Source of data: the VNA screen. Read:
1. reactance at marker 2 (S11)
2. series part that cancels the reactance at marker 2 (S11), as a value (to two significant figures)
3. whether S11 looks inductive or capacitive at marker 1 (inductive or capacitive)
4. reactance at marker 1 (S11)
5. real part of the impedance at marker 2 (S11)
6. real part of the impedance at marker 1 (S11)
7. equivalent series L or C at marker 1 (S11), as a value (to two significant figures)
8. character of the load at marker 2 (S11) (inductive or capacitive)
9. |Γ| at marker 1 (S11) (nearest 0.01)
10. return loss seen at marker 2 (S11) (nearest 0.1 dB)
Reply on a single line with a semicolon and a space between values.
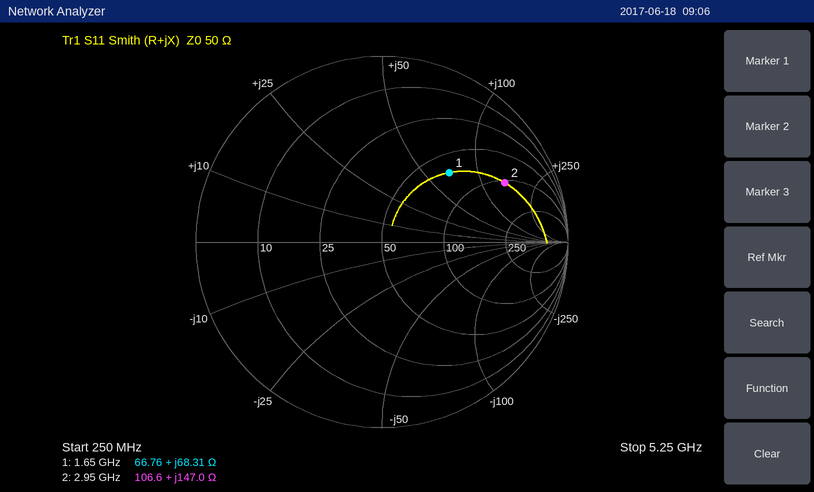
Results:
+147.0 Ω; 370 fF; inductive; +68.31 Ω; 106.6 Ω; 66.76 Ω; 6.6 nH; inductive; 0.52; 2.7 dB
